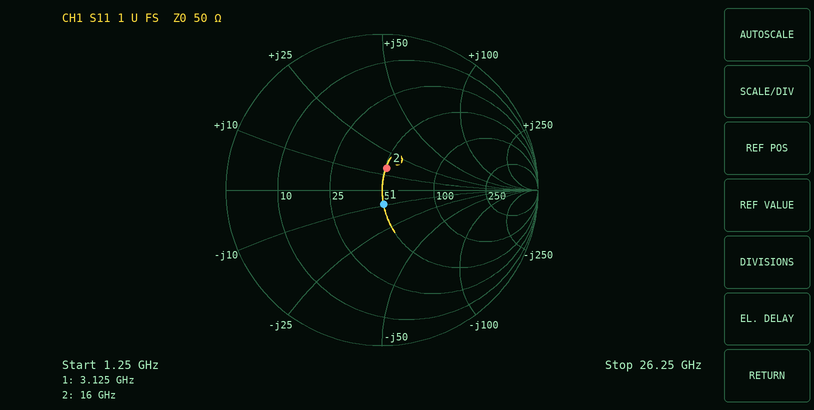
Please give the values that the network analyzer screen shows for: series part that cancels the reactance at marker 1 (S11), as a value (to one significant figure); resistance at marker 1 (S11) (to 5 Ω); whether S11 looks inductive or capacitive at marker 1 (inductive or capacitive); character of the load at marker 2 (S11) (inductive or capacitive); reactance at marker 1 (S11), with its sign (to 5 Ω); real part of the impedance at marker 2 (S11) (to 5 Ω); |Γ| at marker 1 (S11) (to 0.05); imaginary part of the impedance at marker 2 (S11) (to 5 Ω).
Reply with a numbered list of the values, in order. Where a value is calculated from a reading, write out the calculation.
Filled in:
1. L = 10 Ω/(2π × 3.125 GHz) ≈ 509 pH, so 500 pH to one significant figure
2. 50 Ω
3. capacitive
4. inductive
5. -10 Ω
6. 50 Ω
7. 0.10
8. +15 Ω
